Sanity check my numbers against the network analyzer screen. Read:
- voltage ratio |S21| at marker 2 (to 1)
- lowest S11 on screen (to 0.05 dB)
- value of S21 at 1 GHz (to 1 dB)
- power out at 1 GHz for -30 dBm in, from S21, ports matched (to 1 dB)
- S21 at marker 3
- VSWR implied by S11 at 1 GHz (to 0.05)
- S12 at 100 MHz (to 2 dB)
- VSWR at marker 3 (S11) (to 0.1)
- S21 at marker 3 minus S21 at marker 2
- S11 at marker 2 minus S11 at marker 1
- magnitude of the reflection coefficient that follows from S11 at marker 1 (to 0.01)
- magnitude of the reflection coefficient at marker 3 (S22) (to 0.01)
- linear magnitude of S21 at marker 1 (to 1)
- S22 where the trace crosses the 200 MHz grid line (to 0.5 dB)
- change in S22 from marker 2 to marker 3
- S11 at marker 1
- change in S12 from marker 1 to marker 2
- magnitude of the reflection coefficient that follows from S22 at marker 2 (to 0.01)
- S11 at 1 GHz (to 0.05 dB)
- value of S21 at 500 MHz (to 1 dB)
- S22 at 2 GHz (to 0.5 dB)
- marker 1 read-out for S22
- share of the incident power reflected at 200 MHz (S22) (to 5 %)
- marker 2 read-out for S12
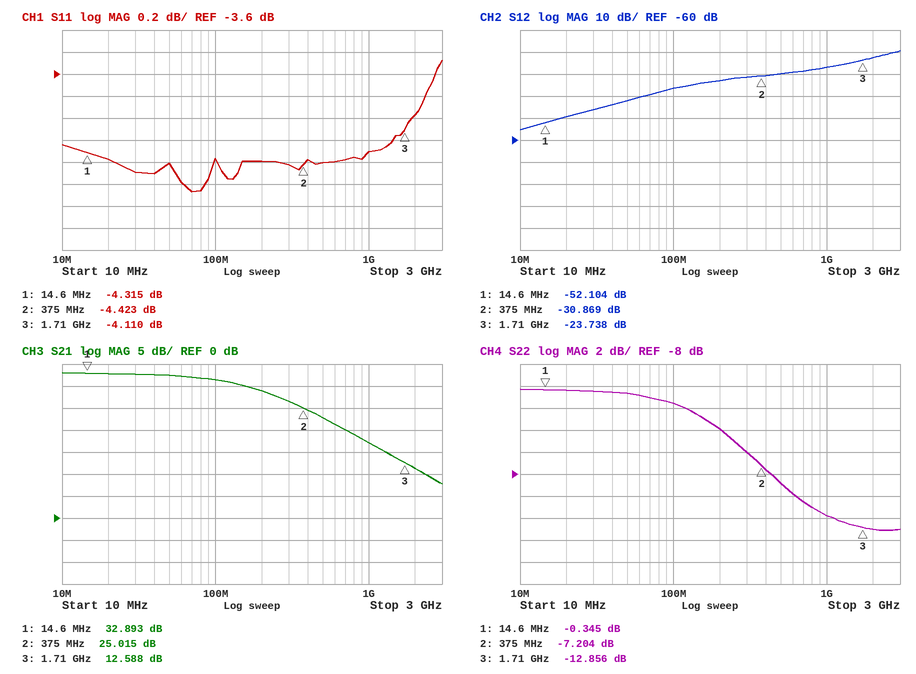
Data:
18
-4.65 dB
17 dB
-13 dBm
12.588 dB
4.10
-36 dB
4.3
-12.427 dB
-0.108 dB
0.61
0.23
44
-4.0 dB
-5.652 dB
-4.315 dB
21.235 dB
0.44
-4.30 dB
23 dB
-13.0 dB
-0.345 dB
40 %
-30.869 dB
